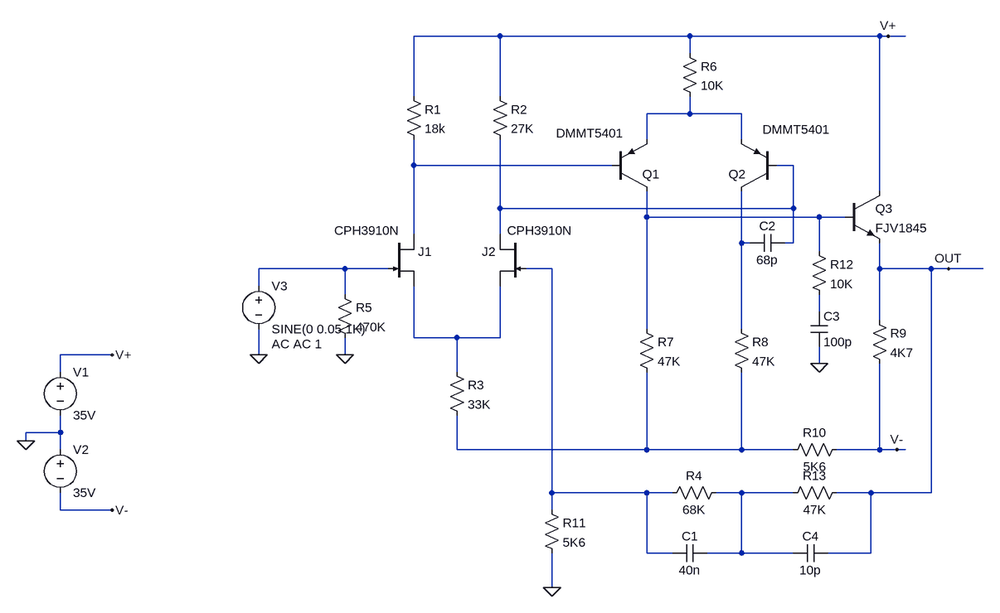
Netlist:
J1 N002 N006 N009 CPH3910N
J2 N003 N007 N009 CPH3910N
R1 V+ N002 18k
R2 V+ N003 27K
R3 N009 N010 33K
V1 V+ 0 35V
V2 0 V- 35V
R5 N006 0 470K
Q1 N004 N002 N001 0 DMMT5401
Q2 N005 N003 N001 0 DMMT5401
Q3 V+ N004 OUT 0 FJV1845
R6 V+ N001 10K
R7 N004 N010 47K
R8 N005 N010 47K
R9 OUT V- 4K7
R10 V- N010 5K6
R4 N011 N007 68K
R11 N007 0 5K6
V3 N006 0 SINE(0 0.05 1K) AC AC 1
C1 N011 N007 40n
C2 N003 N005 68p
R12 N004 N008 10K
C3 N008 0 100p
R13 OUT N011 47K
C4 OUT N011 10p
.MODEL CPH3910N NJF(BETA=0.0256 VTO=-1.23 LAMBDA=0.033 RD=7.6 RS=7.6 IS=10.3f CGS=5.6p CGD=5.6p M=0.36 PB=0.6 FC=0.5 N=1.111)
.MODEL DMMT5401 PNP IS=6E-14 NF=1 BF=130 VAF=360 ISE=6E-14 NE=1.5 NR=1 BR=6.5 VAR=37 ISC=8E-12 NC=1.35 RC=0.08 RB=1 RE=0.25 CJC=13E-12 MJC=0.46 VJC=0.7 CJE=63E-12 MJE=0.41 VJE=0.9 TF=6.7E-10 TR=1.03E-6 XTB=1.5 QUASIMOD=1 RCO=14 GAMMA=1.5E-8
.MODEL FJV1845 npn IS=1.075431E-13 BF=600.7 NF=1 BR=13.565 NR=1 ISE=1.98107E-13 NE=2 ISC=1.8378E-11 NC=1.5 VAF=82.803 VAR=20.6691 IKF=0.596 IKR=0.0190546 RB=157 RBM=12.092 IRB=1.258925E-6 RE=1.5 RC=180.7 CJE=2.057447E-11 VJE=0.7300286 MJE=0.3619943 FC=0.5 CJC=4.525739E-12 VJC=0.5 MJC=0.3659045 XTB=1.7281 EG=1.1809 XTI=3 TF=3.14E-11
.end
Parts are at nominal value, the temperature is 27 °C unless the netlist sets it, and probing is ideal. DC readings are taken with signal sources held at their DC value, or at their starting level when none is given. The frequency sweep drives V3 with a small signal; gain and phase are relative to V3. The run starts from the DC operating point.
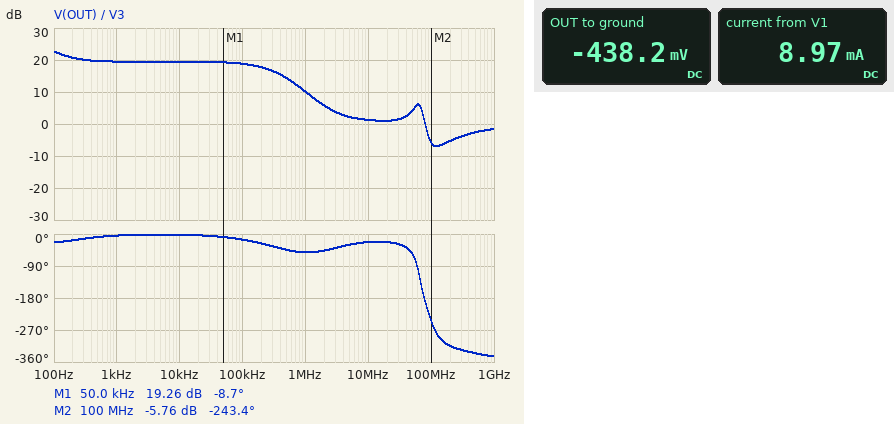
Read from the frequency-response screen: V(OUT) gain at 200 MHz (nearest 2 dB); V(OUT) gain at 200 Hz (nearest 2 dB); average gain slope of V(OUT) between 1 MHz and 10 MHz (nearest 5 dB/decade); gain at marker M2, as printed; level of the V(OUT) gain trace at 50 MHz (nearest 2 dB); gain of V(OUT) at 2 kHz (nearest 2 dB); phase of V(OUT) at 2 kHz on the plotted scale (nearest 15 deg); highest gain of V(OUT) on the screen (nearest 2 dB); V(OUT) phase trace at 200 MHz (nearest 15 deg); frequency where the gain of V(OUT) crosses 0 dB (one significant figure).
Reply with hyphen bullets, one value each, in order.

- -6 dB
- 20 dB
- -10 dB/decade
- -5.76 dB
- 4 dB
- 20 dB
- 0 deg
- 22 dB
- -315 deg
- 80 MHz
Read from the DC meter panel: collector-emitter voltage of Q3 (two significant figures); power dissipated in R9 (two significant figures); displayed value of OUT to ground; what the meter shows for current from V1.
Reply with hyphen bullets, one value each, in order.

- 35 V
- 250 mW
- -438.2 mV
- 8.97 mA
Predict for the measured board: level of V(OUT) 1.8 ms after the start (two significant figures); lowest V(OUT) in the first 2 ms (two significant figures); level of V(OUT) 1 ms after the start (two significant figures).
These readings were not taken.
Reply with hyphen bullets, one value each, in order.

- -880 mV
- -890 mV
- -450 mV
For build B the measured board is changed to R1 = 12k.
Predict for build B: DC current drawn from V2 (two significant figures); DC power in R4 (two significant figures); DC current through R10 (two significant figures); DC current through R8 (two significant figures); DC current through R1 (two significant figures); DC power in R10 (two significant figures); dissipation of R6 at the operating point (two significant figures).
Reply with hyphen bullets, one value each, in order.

- 8.7 mA
- 3.4 µW
- 1.5 mA
- 62 µA
- 580 µA
- 12 mW
- 4.1 mW
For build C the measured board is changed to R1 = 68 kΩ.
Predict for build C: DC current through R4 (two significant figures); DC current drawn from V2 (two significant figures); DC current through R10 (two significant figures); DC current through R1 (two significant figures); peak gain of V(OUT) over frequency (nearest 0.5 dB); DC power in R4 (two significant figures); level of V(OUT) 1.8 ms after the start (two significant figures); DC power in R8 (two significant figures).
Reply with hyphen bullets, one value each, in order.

- 7.8 µA
- 9.7 mA
- 2.1 mA
- 210 µA
- 26.5 dB
- 4.1 µW
- 500 mV
- 30 mW
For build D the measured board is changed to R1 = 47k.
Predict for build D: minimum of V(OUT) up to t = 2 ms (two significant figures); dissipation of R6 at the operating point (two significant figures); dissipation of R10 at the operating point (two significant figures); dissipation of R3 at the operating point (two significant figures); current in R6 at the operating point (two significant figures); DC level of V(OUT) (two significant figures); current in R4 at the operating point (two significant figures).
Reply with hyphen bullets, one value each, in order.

- 130 mV
- 15 mW
- 22 mW
- 19 mW
- 1.2 mA
- 580 mV
- 4.8 µA
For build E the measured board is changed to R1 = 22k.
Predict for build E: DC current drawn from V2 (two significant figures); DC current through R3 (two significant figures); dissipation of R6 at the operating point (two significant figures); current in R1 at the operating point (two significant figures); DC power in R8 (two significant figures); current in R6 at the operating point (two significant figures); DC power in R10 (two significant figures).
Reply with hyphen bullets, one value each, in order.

- 9.1 mA
- 810 µA
- 8.3 mW
- 440 µA
- 5.5 mW
- 910 µA
- 16 mW
